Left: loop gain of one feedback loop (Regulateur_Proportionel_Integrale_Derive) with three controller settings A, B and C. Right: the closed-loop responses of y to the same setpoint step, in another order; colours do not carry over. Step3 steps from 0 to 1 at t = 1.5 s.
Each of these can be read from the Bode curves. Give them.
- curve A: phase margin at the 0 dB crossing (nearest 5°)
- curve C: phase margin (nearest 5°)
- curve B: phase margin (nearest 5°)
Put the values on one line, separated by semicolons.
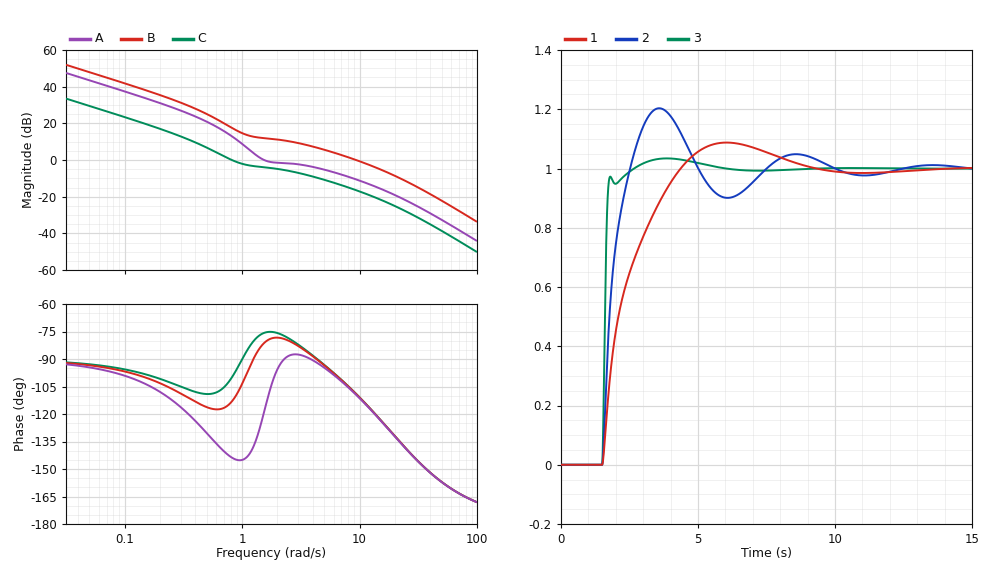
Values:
60°; 80°; 70°
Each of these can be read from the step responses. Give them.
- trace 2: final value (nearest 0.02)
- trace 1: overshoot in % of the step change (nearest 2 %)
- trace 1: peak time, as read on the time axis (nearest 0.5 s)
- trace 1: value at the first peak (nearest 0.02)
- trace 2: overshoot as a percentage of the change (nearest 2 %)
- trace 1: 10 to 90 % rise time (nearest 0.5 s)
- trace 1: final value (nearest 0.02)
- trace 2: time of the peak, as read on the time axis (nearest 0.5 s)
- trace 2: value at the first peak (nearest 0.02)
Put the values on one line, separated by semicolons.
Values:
1.00; 8 %; 6.0 s; 1.08; 20 %; 2.0 s; 1.00; 3.5 s; 1.20
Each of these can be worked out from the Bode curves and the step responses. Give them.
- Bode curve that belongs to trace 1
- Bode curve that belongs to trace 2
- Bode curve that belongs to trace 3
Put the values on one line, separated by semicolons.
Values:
C; A; B
